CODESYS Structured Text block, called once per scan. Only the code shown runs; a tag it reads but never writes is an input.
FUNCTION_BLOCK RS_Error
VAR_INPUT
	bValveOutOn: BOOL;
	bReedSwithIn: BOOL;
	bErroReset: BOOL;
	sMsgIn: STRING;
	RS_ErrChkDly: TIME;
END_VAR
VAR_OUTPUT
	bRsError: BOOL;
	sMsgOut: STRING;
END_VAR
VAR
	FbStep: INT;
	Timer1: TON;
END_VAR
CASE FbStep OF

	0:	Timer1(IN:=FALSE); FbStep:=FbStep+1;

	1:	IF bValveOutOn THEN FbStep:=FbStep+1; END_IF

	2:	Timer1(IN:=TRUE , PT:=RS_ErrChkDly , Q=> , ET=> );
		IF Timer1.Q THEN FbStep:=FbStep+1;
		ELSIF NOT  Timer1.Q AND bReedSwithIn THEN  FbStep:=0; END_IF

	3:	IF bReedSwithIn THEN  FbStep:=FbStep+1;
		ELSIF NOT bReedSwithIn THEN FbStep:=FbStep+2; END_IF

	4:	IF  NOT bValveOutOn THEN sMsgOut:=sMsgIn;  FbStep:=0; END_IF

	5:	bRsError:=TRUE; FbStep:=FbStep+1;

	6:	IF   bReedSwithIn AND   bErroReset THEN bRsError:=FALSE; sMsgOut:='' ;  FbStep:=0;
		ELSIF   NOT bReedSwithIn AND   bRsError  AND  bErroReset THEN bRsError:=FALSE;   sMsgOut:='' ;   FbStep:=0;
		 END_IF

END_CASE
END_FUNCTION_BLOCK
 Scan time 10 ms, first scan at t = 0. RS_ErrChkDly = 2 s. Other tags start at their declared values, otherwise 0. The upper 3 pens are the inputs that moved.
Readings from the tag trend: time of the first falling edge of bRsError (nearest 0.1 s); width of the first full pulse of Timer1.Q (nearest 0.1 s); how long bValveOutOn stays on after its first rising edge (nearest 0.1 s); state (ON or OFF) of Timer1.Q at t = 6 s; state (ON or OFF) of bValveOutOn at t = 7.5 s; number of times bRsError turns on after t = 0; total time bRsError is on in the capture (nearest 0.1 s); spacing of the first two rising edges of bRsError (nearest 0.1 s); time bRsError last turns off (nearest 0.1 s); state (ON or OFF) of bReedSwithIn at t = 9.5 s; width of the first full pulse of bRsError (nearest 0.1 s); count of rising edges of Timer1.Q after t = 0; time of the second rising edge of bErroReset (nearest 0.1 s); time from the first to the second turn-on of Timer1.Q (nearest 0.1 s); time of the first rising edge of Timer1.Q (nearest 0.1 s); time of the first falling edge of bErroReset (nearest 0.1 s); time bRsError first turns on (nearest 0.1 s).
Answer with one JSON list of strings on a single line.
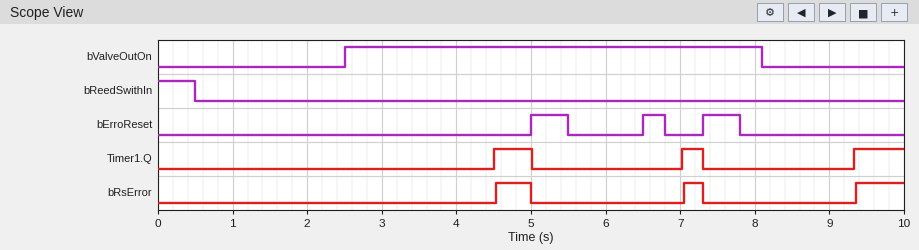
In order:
["5.0 s", "0.5 s", "5.6 s", "OFF", "ON", "3", "1.4 s", "2.5 s", "7.3 s", "OFF", "0.5 s", "3", "6.5 s", "2.5 s", "4.5 s", "5.5 s", "4.5 s"]
